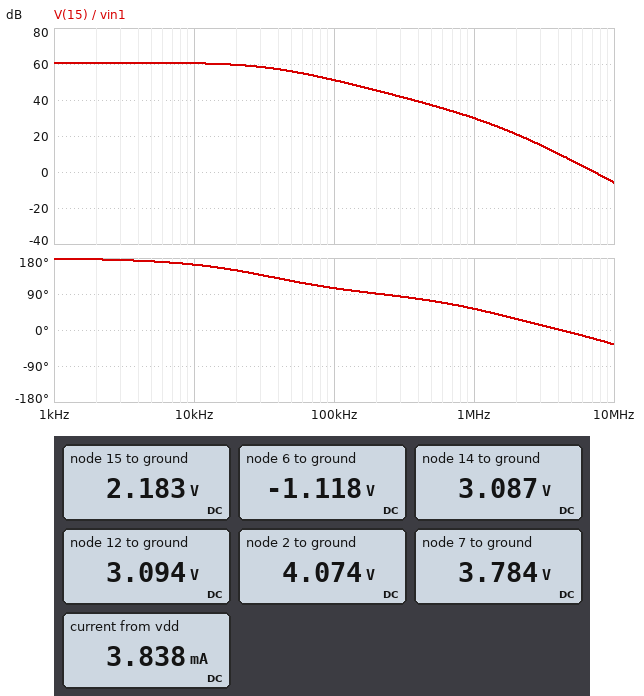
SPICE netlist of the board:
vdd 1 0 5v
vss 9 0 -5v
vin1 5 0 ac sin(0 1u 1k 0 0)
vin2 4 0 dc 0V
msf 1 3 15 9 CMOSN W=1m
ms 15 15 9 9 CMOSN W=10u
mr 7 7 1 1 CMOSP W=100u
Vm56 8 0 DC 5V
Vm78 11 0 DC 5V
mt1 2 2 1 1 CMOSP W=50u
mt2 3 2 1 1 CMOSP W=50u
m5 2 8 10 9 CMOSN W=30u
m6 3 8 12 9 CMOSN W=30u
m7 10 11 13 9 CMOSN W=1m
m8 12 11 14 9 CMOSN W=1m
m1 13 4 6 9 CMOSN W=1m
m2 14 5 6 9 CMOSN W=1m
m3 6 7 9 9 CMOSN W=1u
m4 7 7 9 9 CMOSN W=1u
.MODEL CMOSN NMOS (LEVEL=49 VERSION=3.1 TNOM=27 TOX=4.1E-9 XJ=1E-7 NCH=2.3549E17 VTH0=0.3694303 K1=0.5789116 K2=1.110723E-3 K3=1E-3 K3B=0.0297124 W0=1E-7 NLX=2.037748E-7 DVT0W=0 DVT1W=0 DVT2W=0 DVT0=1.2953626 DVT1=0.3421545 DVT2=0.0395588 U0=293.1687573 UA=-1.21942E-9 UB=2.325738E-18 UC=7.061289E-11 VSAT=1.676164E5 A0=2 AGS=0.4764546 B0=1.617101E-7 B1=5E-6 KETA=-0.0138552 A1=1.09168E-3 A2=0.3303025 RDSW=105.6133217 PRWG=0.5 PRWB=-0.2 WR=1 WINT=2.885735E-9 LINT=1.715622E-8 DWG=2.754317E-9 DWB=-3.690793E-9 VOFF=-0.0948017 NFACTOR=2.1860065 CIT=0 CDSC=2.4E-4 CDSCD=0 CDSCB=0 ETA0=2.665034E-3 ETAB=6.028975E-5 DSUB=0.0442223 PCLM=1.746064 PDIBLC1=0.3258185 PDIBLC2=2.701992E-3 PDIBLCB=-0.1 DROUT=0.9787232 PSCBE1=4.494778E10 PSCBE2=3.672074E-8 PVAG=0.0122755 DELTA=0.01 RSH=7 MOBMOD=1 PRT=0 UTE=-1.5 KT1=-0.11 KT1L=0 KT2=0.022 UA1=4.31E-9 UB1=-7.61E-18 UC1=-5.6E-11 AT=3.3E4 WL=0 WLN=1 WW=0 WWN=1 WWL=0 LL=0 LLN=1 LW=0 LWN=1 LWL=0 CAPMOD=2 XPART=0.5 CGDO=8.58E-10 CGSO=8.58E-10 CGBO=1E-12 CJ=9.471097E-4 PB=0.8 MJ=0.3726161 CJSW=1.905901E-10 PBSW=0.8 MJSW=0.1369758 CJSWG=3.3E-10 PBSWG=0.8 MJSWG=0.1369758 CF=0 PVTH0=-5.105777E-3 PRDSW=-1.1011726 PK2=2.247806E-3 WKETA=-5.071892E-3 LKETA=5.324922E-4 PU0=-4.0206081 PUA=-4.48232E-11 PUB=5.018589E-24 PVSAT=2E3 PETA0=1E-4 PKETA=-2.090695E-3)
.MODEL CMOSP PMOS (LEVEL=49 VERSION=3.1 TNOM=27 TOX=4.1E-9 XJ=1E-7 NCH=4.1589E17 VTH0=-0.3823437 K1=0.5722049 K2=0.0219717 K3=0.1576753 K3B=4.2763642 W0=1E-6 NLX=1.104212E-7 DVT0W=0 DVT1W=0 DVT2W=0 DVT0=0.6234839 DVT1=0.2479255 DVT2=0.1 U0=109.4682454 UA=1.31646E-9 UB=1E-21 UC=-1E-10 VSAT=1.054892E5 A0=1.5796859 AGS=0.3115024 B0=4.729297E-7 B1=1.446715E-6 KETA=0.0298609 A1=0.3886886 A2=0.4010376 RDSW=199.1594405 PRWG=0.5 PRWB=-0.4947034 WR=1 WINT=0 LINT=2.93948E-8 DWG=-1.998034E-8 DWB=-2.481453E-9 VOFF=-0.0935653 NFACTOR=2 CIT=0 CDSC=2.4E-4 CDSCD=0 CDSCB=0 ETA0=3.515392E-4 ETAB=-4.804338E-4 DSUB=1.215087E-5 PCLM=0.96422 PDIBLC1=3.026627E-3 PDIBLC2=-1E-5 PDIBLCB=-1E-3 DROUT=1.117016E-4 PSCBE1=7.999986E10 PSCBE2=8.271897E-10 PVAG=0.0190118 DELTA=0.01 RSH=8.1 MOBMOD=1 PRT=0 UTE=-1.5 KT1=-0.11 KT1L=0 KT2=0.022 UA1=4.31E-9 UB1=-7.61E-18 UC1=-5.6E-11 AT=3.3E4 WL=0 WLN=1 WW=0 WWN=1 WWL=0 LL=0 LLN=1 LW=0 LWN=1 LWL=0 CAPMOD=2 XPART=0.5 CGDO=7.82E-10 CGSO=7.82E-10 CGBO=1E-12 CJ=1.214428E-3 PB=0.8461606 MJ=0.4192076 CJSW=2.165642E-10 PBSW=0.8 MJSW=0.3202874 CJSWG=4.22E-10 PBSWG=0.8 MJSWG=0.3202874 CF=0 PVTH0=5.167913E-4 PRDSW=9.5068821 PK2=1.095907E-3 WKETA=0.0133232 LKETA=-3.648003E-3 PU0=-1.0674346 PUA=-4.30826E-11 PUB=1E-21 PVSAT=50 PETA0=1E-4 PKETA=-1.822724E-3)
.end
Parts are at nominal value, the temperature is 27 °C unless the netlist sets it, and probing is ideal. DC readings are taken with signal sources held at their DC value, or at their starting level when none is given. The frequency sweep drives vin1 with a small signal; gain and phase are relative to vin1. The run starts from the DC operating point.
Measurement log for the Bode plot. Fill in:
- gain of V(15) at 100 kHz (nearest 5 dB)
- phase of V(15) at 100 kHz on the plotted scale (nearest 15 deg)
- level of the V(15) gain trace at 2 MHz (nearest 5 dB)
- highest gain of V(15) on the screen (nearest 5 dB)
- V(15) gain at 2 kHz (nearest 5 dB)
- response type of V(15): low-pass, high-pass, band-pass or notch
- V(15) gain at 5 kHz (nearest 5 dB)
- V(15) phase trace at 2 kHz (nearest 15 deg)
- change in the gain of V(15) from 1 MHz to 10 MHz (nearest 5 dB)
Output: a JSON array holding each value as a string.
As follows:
["50 dB", "105 deg", "20 dB", "60 dB", "60 dB", "low-pass", "60 dB", "180 deg", "-35 dB"]
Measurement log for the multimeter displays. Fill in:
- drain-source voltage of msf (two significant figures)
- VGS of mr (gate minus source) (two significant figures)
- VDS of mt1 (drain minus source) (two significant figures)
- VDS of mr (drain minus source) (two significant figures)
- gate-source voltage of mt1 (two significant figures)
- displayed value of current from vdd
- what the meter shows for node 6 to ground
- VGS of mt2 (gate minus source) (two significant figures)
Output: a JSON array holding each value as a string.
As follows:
["2.8 V", "-1.2 V", "-930 mV", "-1.2 V", "-930 mV", "3.838 mA", "-1.118 V", "-930 mV"]
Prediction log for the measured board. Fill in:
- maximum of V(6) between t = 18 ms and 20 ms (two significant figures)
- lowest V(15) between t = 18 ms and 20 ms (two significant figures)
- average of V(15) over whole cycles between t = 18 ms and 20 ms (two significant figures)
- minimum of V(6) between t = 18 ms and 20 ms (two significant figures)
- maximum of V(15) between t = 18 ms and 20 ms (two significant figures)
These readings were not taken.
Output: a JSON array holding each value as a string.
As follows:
["-1.1 V", "2.2 V", "2.2 V", "-1.1 V", "2.2 V"]
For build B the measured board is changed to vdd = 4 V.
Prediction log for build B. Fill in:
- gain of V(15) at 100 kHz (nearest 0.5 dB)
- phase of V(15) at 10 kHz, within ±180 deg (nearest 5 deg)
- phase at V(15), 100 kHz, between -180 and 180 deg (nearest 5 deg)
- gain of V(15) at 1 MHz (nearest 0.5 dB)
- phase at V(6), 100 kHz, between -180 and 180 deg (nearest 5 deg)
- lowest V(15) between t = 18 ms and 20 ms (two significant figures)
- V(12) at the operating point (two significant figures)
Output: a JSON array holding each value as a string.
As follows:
["35.0 dB", "145 deg", "95 deg", "13.0 dB", "5 deg", "1.3 V", "2.9 V"]
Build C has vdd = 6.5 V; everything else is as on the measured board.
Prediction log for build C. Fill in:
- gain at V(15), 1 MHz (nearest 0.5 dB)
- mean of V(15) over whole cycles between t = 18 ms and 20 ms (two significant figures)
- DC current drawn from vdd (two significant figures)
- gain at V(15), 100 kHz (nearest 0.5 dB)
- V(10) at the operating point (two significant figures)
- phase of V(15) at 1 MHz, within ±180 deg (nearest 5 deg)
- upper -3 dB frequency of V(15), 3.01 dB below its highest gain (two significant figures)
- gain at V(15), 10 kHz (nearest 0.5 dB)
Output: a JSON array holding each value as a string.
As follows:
["29.0 dB", "3.6 V", "3.9 mA", "50.5 dB", "3.1 V", "50 deg", "33 kHz", "60.0 dB"]
